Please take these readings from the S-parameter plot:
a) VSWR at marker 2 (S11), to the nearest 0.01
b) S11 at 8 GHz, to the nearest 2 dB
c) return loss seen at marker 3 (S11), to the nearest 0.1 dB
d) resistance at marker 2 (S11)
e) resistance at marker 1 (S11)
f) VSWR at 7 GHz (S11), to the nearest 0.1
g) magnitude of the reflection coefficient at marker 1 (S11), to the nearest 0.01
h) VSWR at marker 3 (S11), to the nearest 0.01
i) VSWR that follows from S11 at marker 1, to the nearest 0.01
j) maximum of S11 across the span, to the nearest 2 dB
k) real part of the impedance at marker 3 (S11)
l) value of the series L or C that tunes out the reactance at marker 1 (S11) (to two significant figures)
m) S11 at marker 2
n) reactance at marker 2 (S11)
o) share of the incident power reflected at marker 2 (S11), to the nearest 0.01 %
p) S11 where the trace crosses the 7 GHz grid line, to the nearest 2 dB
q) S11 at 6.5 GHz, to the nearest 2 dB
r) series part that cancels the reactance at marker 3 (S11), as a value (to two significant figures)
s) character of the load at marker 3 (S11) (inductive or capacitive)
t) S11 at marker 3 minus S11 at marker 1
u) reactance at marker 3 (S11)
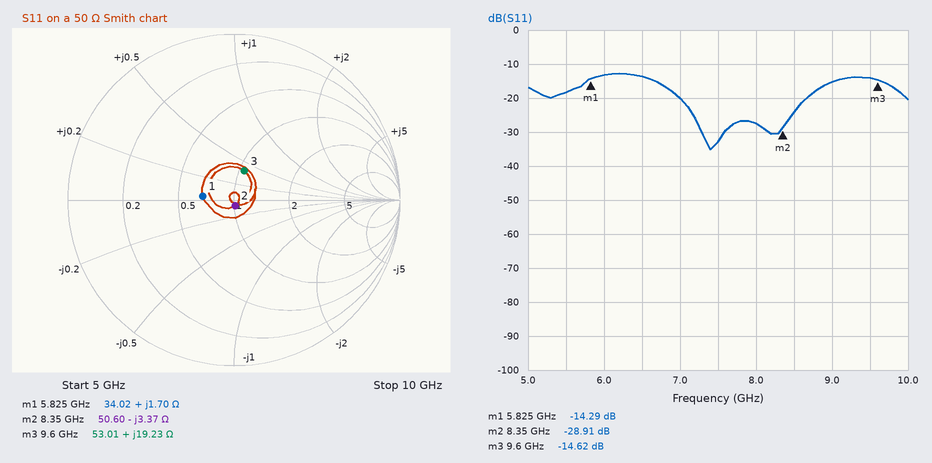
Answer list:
1.07
-28 dB
14.6 dB
50.60 Ω
34.02 Ω
1.2
0.19
1.46
1.48
-12 dB
53.01 Ω
16 pF
-28.91 dB
-3.37 Ω
0.13 %
-20 dB
-14 dB
860 fF
inductive
-0.33 dB
+19.23 Ω
